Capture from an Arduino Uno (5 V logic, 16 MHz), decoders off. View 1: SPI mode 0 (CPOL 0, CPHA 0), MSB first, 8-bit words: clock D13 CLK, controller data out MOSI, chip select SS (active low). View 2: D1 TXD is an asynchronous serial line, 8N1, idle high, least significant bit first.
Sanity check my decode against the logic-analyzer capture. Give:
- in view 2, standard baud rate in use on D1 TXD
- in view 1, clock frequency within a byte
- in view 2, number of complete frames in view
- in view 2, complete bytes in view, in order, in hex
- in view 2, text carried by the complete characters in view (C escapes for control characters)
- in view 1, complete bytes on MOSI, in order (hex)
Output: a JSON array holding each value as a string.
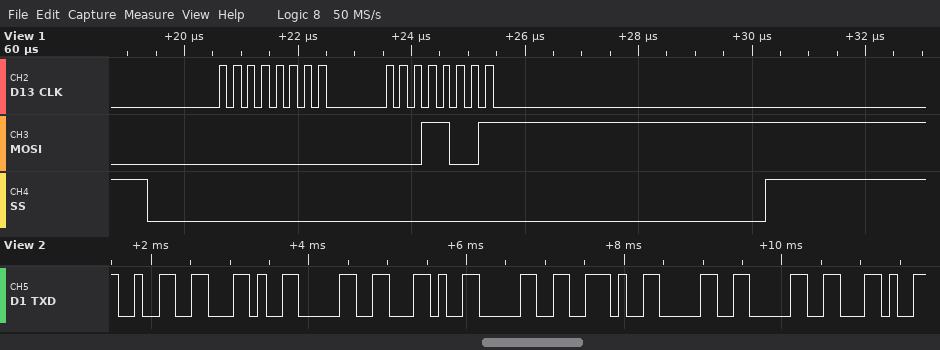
["9600 baud", "4 MHz", "9", "0x32 0x2C 0x30 0x2C 0x30 0x2E 0x30 0x30 0x2C", "\"2,0,0.00,\"", "00 19"]
